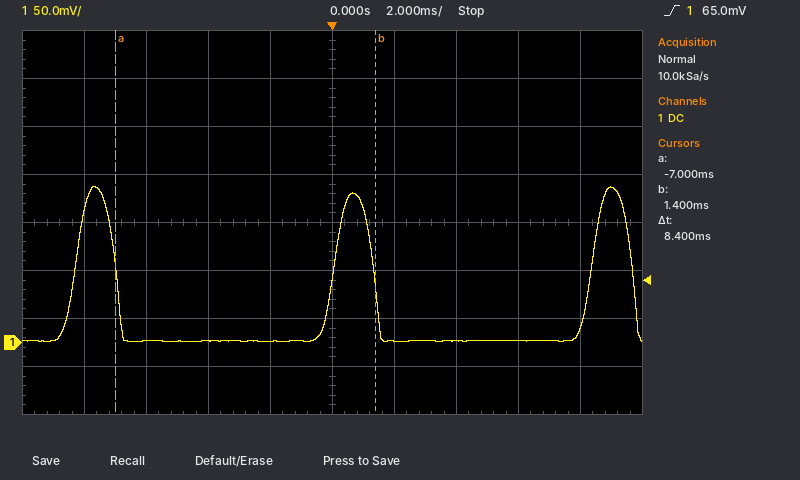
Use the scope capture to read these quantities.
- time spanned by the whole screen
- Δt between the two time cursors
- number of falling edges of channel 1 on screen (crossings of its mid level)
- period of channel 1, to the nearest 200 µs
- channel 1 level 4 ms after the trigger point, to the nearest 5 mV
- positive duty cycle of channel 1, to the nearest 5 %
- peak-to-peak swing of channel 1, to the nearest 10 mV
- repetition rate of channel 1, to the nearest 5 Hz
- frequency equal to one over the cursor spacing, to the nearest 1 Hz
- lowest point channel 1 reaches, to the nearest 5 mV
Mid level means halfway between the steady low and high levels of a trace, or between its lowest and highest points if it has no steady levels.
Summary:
20 ms
8.4 ms
3
8.4 ms
0 mV
15 %
160 mV
120 Hz
119 Hz
0 mV
